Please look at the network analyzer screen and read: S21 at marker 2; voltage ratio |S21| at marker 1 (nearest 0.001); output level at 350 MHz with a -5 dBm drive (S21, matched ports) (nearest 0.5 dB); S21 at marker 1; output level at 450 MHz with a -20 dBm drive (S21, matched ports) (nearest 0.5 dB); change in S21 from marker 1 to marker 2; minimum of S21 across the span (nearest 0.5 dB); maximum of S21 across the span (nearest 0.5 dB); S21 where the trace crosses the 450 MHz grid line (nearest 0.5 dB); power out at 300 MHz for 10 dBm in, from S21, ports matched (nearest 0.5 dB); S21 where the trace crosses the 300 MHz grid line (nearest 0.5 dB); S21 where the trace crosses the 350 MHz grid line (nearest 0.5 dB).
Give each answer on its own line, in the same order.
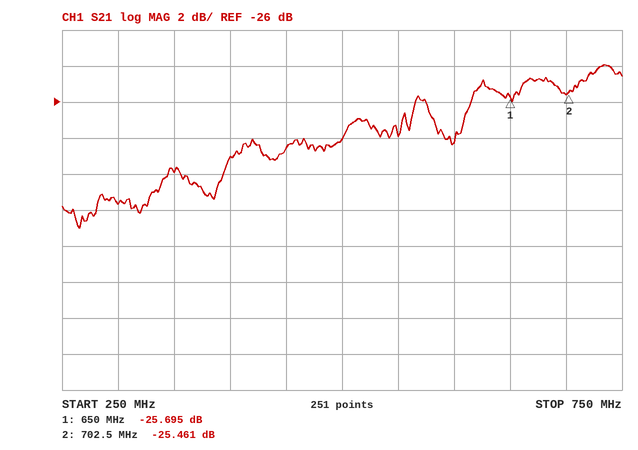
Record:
-25.461 dB
0.052
-35.0 dBm
-25.695 dB
-48.5 dBm
0.234 dB
-33.0 dB
-24.0 dB
-28.5 dB
-21.5 dBm
-31.5 dB
-30.0 dB
